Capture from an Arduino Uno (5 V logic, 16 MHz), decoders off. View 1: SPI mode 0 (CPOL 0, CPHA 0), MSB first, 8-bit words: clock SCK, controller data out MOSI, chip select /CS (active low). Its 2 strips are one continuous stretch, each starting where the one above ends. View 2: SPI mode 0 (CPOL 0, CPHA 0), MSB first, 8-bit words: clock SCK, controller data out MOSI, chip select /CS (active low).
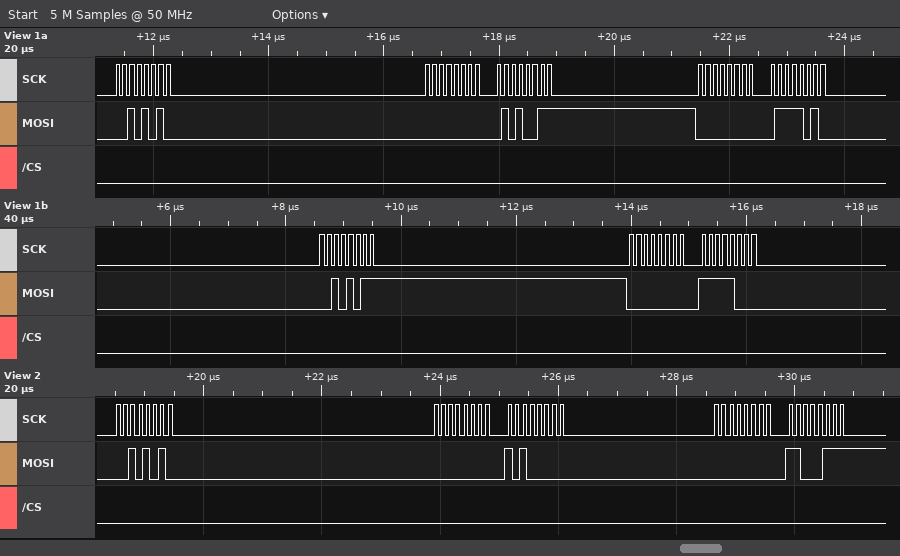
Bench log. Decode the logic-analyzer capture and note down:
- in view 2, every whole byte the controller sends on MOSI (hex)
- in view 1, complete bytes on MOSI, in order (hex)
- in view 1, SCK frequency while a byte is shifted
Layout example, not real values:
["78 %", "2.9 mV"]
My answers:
["2A 00 A0 00 C7", "0x2A 0x00 0x53 0x00 0x7A 0x2B 0x00 0xF8", "8 MHz"]
